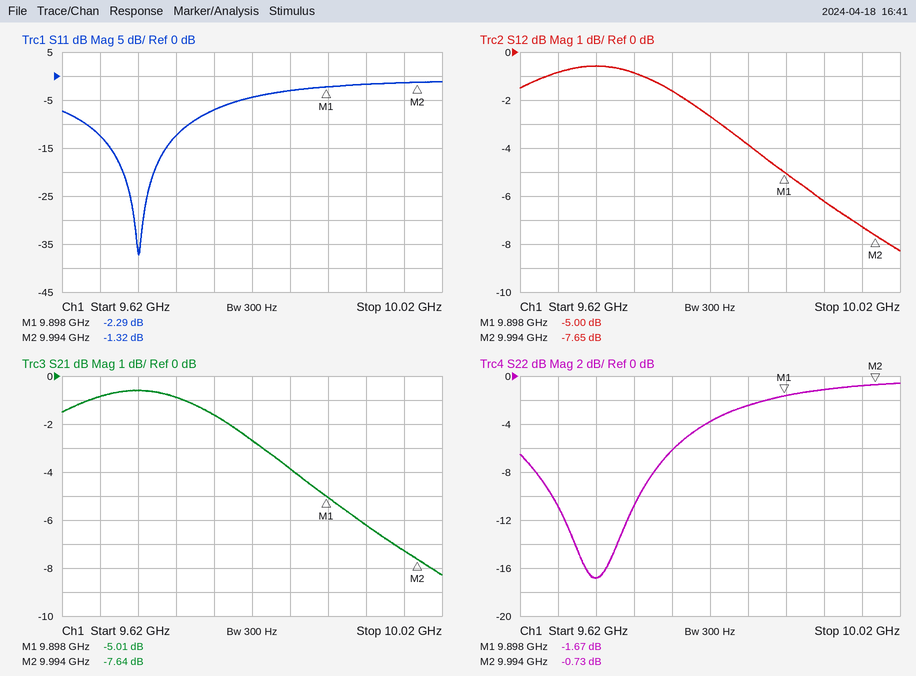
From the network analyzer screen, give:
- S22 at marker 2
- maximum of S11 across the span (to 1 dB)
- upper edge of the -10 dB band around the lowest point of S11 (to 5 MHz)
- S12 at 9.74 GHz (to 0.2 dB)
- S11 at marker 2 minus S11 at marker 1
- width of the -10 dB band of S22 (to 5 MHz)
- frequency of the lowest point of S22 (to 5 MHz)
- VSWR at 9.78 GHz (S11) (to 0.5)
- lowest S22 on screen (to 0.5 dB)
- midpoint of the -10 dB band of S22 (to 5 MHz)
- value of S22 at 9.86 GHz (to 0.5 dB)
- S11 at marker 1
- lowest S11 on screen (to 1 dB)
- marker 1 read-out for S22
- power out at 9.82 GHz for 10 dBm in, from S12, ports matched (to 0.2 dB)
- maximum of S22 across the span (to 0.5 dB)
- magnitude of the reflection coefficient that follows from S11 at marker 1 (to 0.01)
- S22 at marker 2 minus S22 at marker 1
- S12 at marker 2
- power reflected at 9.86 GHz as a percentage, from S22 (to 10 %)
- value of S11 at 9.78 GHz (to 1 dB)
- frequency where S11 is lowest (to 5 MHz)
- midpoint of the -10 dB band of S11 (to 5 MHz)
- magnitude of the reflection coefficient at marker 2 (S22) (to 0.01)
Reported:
-0.73 dB
-1 dB
9.755 GHz
-0.8 dB
0.97 dB
90 MHz
9.700 GHz
2.5
-17.0 dB
9.700 GHz
-2.5 dB
-2.29 dB
-37 dB
-1.67 dB
7.4 dBm
-0.5 dB
0.77
0.94 dB
-7.65 dB
60 %
-7 dB
9.700 GHz
9.700 GHz
0.92
